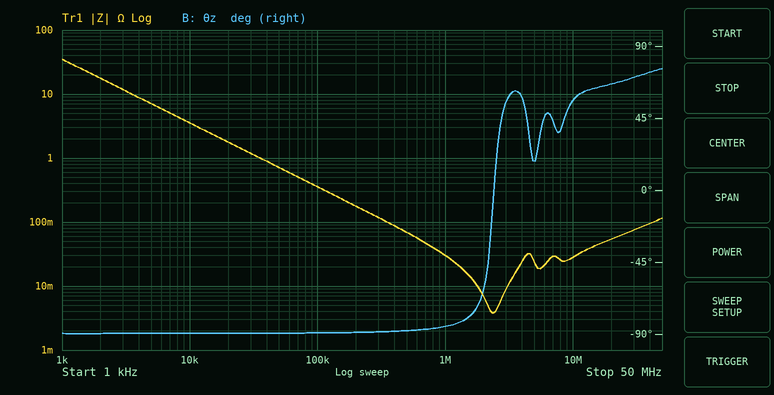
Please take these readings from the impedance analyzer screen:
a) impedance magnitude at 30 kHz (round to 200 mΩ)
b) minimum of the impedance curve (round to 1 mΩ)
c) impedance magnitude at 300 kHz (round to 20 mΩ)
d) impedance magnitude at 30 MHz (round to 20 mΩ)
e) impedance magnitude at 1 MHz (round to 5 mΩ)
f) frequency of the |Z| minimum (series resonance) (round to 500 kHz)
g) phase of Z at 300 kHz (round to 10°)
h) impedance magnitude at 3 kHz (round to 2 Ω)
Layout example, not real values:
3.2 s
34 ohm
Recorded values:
1.2 Ω
4 mΩ
120 mΩ
80 mΩ
30 mΩ
2.5 MHz
-90°
12 Ω
